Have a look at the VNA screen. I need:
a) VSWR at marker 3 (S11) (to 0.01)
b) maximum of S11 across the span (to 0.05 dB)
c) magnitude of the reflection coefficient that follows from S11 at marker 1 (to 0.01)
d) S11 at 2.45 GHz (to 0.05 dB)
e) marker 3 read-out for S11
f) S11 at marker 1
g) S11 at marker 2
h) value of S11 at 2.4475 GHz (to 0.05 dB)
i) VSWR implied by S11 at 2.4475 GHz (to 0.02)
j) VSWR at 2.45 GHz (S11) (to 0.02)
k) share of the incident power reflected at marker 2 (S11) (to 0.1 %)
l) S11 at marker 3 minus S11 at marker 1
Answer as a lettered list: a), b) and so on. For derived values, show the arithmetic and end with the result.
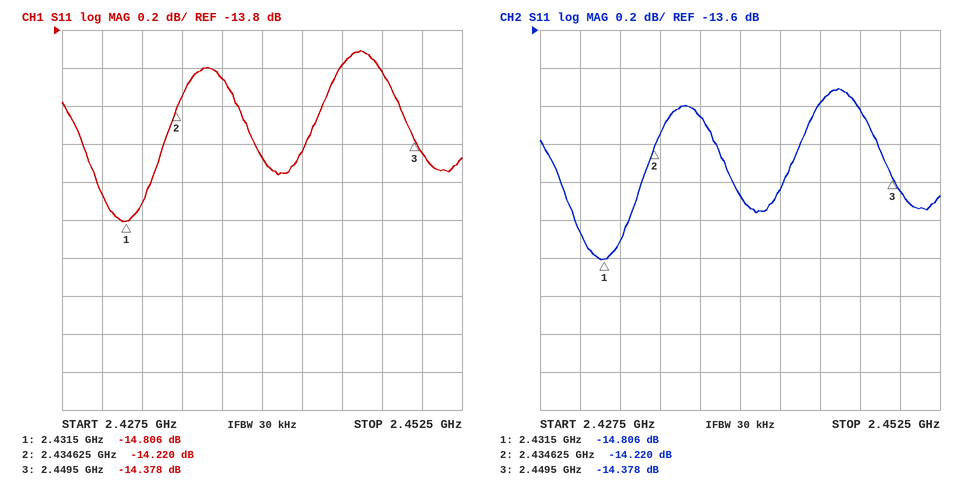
a) (1 + 0.1910)/(1 − 0.1910) ≈ 1.47
b) -13.90 dB
c) 10^(-14.806/20) ≈ 0.18
d) -14.45 dB
e) -14.378 dB
f) -14.806 dB
g) -14.220 dB
h) -14.00 dB
i) |Γ| = 10^(-14/20) = 0.1995; VSWR = (1 + 0.1995)/(1 − 0.1995) ≈ 1.50
j) |Γ| = 10^(-14.45/20) = 0.1895; VSWR = (1 + 0.1895)/(1 − 0.1895) ≈ 1.47, so 1.46 to the nearest 0.02
k) 10^(-14.22/10) ≈ 3.8 %
l) -14.378 − (-14.806) = 0.428 dB
